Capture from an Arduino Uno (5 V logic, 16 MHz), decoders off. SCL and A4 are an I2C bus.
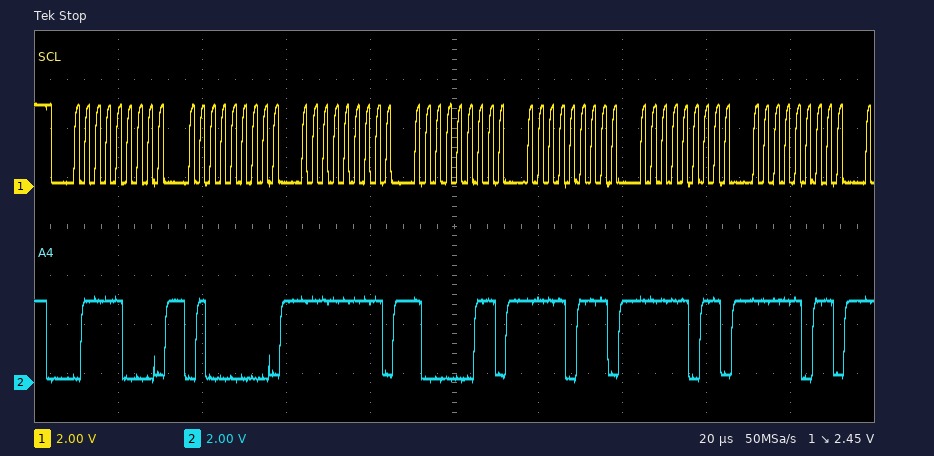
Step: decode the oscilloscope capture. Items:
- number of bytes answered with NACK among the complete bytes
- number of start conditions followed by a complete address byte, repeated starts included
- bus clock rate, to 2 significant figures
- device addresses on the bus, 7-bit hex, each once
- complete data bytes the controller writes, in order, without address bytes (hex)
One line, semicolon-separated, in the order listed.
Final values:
0; 1; 400 kHz; 0x3C; 40 FF 83 F7 FB FB
